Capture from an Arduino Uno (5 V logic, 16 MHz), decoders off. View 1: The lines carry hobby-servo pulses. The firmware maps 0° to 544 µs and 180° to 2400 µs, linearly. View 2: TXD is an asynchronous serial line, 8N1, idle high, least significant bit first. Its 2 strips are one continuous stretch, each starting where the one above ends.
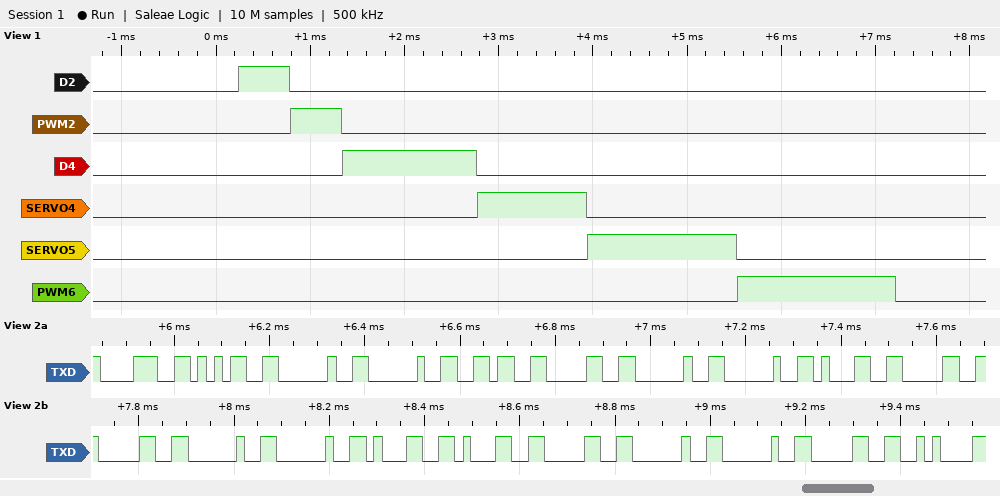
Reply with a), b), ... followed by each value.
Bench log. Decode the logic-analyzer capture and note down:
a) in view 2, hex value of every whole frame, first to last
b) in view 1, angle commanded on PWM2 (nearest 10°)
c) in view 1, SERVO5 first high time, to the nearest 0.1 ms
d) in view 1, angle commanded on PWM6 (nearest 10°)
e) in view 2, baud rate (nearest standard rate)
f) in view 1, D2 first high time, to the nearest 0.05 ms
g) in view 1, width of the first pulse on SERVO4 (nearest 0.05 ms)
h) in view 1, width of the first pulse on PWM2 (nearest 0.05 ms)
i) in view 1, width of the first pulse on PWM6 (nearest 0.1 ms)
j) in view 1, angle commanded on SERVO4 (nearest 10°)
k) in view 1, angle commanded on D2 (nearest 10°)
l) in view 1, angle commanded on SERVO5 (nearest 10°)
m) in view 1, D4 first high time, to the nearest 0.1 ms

a) 38 35 20 20 36 30 20 20 31 30 30 20 20 31 31 30 20 20 30 0A
b) 0°
c) 1.6 ms
d) 110°
e) 57600 baud
f) 0.55 ms
g) 1.15 ms
h) 0.55 ms
i) 1.7 ms
j) 60°
k) 0°
l) 100°
m) 1.4 ms
